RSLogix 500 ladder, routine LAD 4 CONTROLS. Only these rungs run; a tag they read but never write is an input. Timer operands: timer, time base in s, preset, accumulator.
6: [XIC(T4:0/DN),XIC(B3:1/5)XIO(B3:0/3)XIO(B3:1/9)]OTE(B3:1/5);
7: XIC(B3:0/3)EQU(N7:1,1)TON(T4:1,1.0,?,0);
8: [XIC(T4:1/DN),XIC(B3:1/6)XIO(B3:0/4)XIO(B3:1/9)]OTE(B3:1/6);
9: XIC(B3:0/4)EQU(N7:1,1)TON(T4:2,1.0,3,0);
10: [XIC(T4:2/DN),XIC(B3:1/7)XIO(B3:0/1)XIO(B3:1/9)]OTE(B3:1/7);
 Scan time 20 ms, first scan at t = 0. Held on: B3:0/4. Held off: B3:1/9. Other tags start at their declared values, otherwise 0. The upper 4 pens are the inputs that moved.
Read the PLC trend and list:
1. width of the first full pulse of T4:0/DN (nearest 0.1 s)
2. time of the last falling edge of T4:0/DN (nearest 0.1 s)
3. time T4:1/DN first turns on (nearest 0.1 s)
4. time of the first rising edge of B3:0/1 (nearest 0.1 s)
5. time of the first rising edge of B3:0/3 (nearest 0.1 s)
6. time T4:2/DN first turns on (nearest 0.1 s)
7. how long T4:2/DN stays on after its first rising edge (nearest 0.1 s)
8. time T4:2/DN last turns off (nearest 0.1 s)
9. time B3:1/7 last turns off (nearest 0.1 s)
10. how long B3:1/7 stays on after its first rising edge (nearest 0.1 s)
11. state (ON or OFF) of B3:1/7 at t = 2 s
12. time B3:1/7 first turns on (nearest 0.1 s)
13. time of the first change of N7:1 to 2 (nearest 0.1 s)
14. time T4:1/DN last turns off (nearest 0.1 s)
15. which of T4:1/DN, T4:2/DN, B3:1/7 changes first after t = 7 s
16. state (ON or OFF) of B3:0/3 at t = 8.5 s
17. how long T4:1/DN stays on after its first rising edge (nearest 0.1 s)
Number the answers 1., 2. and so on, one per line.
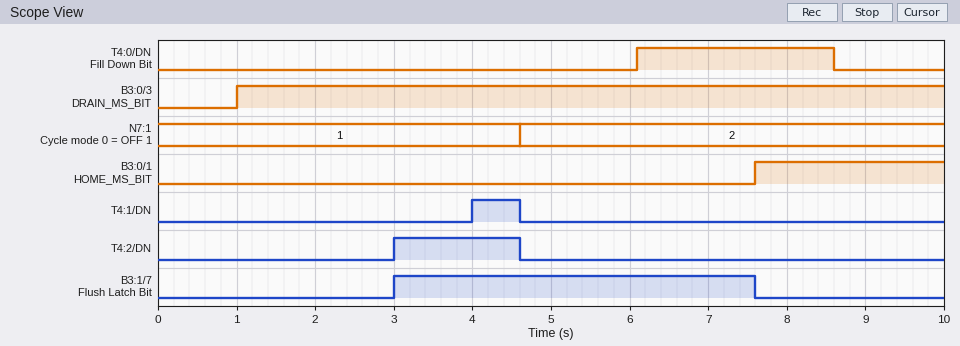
1. 2.5 s
2. 8.6 s
3. 4.0 s
4. 7.6 s
5. 1.0 s
6. 3.0 s
7. 1.6 s
8. 4.6 s
9. 7.6 s
10. 4.6 s
11. OFF
12. 3.0 s
13. 4.6 s
14. 4.6 s
15. B3:1/7
16. ON
17. 0.6 s
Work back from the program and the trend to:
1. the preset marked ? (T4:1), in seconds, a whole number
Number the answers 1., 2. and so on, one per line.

1. 3 s
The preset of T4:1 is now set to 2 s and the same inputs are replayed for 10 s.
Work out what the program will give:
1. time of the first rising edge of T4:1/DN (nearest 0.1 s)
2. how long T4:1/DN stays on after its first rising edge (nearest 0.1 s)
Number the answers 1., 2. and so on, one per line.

1. 3.0 s
2. 1.6 s
